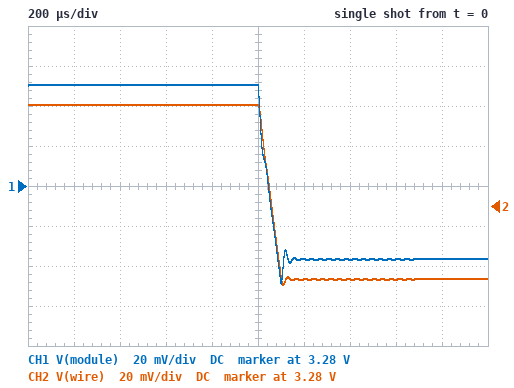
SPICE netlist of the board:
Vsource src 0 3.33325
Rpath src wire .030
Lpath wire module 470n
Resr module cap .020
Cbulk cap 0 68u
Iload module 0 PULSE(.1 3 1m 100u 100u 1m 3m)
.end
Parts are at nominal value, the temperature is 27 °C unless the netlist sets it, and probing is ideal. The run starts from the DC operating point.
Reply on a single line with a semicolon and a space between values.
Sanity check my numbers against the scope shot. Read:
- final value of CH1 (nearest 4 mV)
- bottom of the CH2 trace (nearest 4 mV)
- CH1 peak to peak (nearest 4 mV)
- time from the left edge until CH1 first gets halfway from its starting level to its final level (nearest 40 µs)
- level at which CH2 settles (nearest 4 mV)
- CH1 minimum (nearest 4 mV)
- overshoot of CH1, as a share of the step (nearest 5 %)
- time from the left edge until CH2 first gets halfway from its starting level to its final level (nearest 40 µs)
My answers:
3.244 V; 3.240 V; 100 mV; 1.04 ms; 3.244 V; 3.232 V; 15 %; 1.04 ms
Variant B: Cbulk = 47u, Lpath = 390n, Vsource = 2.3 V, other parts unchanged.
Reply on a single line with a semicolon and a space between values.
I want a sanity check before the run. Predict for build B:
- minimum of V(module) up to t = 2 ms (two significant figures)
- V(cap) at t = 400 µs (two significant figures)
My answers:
2.2 V; 2.3 V
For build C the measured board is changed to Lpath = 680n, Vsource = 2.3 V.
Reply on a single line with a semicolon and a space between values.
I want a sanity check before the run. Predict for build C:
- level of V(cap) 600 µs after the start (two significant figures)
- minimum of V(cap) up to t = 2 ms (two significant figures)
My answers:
2.3 V; 2.2 V
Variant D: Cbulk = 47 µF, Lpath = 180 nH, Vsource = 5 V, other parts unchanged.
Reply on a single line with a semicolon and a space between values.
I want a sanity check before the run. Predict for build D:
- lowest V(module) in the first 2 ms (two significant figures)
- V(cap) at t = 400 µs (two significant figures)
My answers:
4.9 V; 5.0 V
